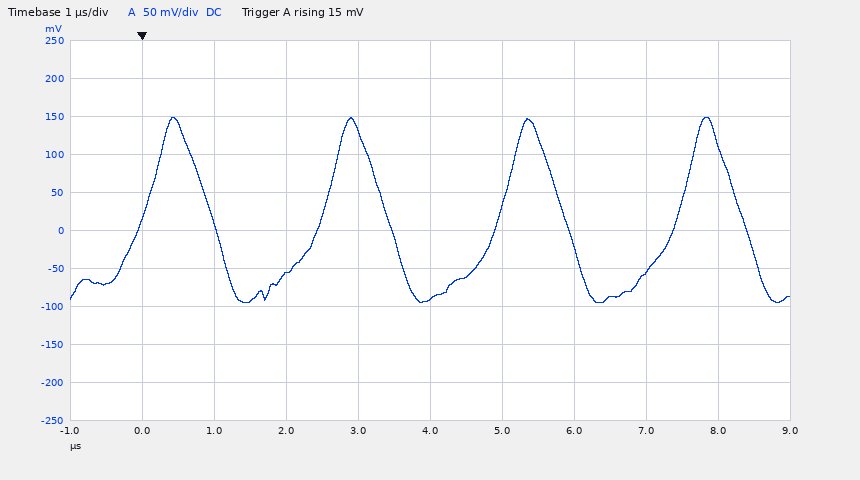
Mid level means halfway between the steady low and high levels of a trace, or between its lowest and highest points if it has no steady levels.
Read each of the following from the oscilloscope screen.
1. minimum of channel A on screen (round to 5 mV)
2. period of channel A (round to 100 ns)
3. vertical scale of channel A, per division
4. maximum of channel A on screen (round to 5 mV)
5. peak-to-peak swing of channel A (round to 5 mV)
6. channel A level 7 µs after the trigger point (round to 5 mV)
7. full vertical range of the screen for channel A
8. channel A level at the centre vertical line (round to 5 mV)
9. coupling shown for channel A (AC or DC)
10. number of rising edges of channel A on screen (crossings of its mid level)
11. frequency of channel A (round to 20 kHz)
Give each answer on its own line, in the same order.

-95 mV
2.5 µs
50 mV
150 mV
245 mV
-55 mV
500 mV
-90 mV
DC
4
400 kHz
